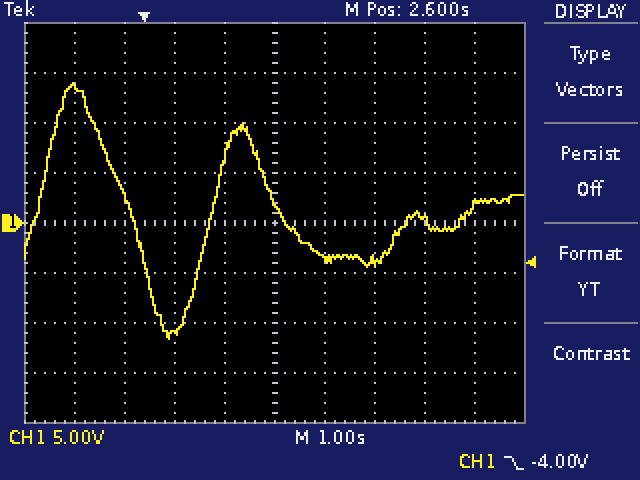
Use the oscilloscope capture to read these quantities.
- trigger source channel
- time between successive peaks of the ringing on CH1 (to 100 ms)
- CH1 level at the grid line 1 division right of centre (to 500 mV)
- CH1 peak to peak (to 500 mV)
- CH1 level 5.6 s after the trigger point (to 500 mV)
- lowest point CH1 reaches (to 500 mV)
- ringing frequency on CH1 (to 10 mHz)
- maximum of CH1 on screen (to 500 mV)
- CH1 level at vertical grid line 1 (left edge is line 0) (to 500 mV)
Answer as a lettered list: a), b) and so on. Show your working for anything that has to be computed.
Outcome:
a) CH1
b) 3.4 s
c) -3.5 V
d) 14.0 V − (-11.5 V) = 25.5 V
e) 500 mV
f) -11.5 V
g) 1 / 3.4 s ≈ 294 mHz, so 290 mHz to the nearest 10 mHz
h) 14.0 V
i) 13.5 V
